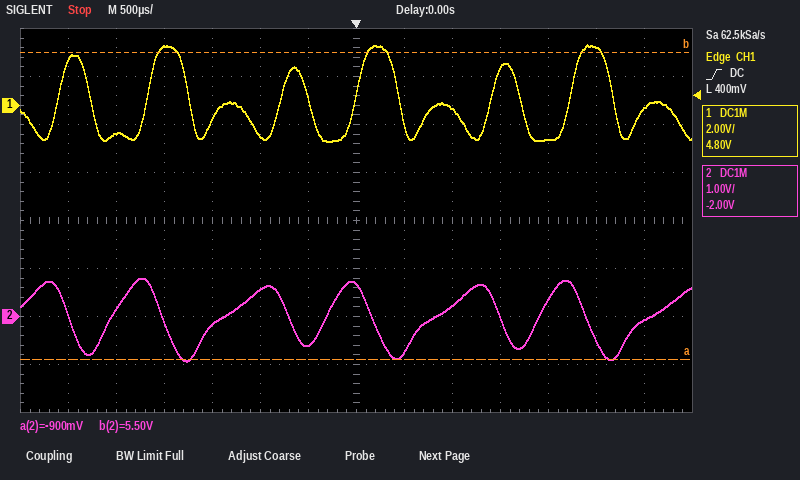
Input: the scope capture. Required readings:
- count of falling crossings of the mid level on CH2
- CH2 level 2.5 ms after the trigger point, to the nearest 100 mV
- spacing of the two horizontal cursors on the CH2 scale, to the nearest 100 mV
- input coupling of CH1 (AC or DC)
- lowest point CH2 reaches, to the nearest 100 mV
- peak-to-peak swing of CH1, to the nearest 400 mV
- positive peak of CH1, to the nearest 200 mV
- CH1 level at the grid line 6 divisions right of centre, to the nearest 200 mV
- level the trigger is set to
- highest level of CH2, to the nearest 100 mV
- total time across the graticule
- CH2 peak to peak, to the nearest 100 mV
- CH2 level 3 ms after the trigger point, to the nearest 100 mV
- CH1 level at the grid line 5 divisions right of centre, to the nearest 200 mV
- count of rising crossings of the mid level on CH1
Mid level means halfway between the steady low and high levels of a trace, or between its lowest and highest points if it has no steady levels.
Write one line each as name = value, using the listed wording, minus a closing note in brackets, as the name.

count of falling crossings of the mid level on CH2 = 6
CH2 level 2.5 ms after the trigger point, to the nearest 100 mV = -500 mV
spacing of the two horizontal cursors on the CH2 scale, to the nearest 100 mV = 6.4 V
input coupling of CH1 = DC
lowest point CH2 reaches, to the nearest 100 mV = -900 mV
peak-to-peak swing of CH1, to the nearest 400 mV = 4.0 V
positive peak of CH1, to the nearest 200 mV = 2.6 V
CH1 level at the grid line 6 divisions right of centre, to the nearest 200 mV = -200 mV
level the trigger is set to = 400 mV
highest level of CH2, to the nearest 100 mV = 800 mV
total time across the graticule = 7 ms
CH2 peak to peak, to the nearest 100 mV = 1.7 V
CH2 level 3 ms after the trigger point, to the nearest 100 mV = -100 mV
CH1 level at the grid line 5 divisions right of centre, to the nearest 200 mV = 2.4 V
count of rising crossings of the mid level on CH1 = 6
